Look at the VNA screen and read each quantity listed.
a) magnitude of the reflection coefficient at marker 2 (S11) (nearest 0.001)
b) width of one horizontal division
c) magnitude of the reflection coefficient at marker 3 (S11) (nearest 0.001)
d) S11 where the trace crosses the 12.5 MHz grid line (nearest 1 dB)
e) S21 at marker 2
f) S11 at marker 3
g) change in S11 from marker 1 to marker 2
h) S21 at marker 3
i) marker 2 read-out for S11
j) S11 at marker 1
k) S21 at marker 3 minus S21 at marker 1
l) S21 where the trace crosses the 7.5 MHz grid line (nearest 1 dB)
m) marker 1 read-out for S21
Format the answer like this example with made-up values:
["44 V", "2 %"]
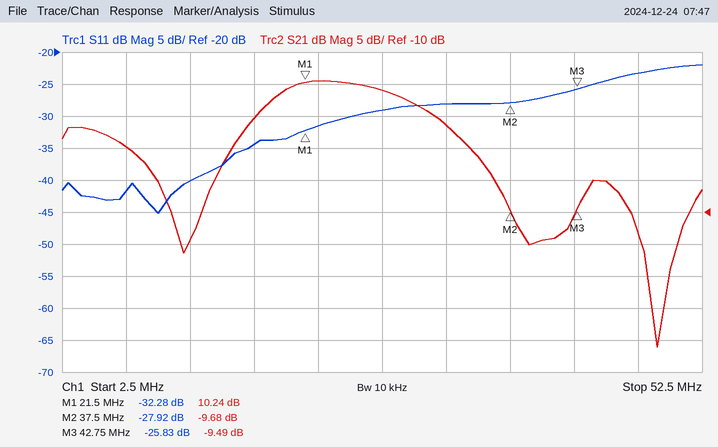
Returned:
["0.040", "5 MHz", "0.051", "-40 dB", "-9.68 dB", "-25.83 dB", "4.36 dB", "-9.49 dB", "-27.92 dB", "-32.28 dB", "-19.73 dB", "0 dB", "10.24 dB"]
